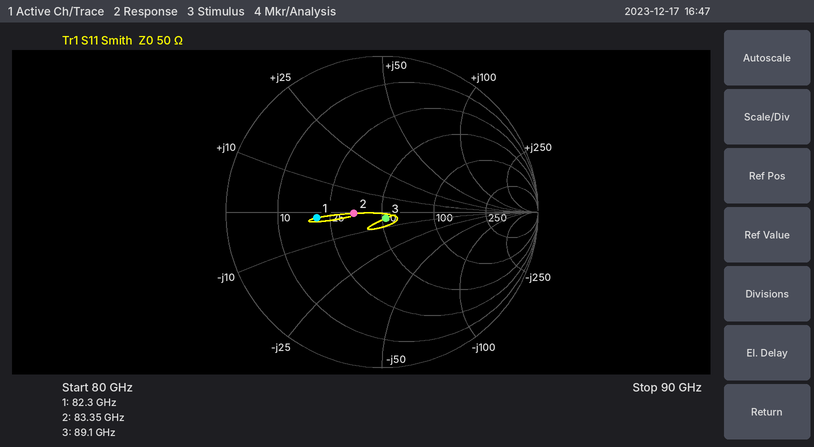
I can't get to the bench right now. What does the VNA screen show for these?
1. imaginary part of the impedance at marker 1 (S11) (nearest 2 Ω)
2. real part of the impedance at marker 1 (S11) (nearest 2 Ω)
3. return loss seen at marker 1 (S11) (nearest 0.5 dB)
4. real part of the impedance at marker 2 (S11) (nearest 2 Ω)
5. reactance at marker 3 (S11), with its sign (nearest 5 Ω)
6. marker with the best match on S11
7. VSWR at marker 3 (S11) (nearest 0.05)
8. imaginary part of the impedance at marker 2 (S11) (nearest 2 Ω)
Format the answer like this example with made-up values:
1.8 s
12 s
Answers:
-2 Ω
20 Ω
7.5 dB
34 Ω
-5 Ω
marker 3
1.10
0 Ω
